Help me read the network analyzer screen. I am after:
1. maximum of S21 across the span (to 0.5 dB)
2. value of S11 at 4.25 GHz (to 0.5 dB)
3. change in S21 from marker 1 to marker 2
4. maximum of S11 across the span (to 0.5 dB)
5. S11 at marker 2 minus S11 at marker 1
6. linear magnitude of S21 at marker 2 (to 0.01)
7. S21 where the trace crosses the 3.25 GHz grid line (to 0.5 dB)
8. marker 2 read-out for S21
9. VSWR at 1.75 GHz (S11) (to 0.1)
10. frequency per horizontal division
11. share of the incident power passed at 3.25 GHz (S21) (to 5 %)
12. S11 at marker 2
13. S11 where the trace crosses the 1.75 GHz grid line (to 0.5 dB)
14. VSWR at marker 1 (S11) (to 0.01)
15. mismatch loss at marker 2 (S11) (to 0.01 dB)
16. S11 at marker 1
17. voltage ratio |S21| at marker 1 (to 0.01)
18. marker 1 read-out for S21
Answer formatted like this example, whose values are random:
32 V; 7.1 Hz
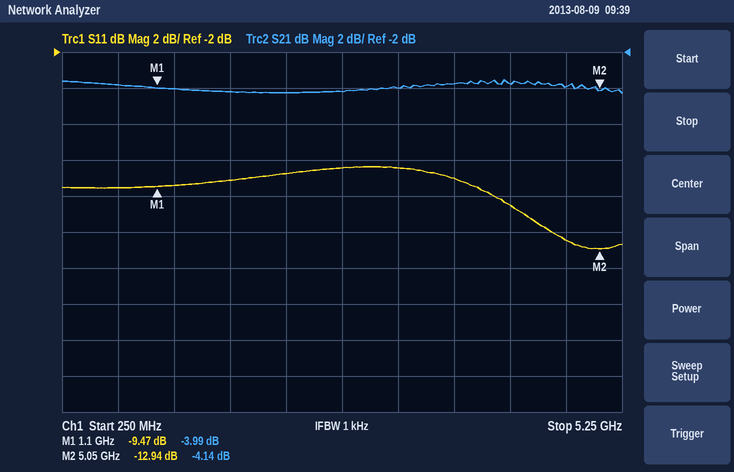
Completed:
-3.5 dB; -10.5 dB; -0.15 dB; -8.5 dB; -3.47 dB; 0.62; -4.0 dB; -4.14 dB; 2.1; 500 MHz; 40 %; -12.94 dB; -9.0 dB; 2.01; 0.23 dB; -9.47 dB; 0.63; -3.99 dB
